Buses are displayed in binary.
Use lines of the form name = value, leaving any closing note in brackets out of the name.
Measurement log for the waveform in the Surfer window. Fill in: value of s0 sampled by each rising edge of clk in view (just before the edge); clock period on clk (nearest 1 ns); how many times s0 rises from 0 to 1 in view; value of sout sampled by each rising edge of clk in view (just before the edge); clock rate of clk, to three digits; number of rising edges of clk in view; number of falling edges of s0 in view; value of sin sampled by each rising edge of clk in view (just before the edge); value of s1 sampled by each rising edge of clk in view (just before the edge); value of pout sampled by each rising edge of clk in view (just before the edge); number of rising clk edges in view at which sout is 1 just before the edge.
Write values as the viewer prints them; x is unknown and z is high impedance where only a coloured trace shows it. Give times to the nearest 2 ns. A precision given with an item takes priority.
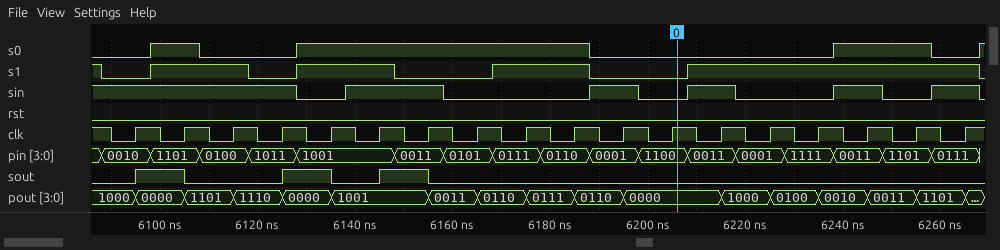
value of s0 sampled by each rising edge of clk in view = 0 1 0 0 1 1 1 1 1 1 0 0 0 0 0 1 1 0
clock period on clk = 10 ns
how many times s0 rises from 0 to 1 in view = 4
value of sout sampled by each rising edge of clk in view = 0 1 0 0 1 0 1 0 0 0 0 0 0 0 0 0 0 0
clock rate of clk, to three digits = 100 MHz
number of rising edges of clk in view = 18
number of falling edges of s0 in view = 3
value of sin sampled by each rising edge of clk in view = 1 1 1 1 0 1 1 0 0 0 1 0 1 0 0 1 0 1
value of s1 sampled by each rising edge of clk in view = 0 1 1 0 1 1 0 0 1 1 0 0 1 1 1 1 1 1
value of pout sampled by each rising edge of clk in view = 1000, 0000, 1101, 1110, 0000, 1001, 1001, 0011, 0110, 0111, 0110, 0000, 0000, 1000, 0100, 0010, 0011, 1101
number of rising clk edges in view at which sout is 1 just before the edge = 3
